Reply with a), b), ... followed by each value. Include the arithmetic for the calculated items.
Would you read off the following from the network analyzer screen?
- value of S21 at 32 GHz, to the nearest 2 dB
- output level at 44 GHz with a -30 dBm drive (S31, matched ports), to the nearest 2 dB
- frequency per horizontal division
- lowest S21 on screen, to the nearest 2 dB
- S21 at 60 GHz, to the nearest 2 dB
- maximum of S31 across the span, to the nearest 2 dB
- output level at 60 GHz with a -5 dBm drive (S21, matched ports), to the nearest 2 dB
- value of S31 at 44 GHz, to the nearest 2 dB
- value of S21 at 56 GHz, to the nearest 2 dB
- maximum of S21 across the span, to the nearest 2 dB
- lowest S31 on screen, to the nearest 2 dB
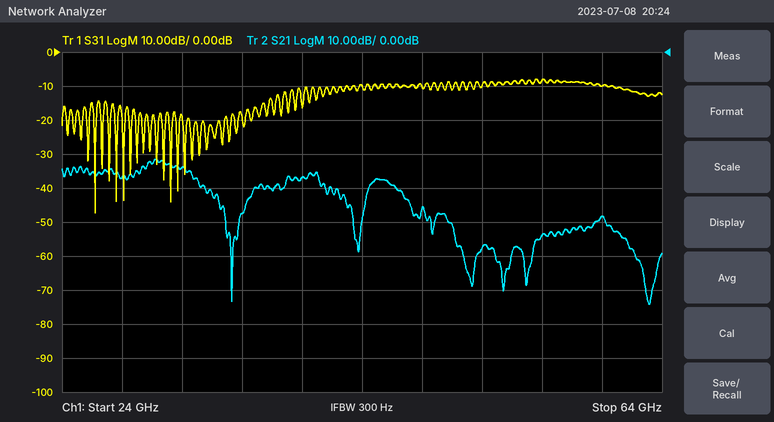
a) -34 dB
b) -30 dBm + (-10 dB) = -40 dBm
c) 4 GHz
d) -74 dB
e) -48 dB
f) -8 dB
g) -5 dBm + (-48 dB) = -54 dBm
h) -10 dB
i) -54 dB
j) -32 dB
k) -48 dB
